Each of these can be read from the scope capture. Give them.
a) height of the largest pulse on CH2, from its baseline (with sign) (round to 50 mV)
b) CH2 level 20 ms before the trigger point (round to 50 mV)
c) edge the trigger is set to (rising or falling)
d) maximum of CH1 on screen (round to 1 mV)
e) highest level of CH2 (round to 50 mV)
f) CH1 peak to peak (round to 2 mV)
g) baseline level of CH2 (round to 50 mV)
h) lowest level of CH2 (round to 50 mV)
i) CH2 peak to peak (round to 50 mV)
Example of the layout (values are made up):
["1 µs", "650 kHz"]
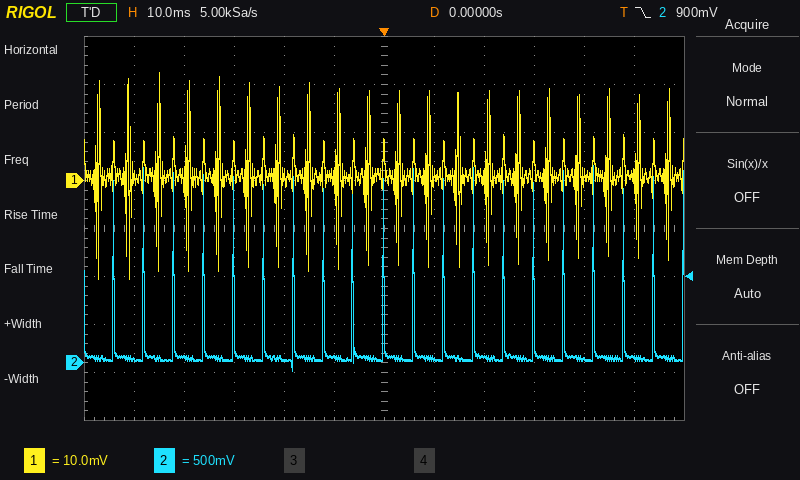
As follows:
["+2.00 V", "50 mV", "falling", "22 mV", "2.05 V", "42 mV", "50 mV", "-100 mV", "2.15 V"]
